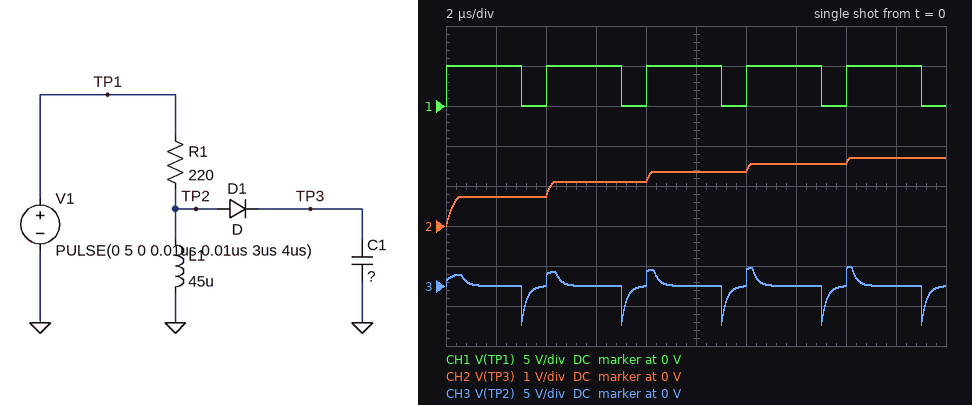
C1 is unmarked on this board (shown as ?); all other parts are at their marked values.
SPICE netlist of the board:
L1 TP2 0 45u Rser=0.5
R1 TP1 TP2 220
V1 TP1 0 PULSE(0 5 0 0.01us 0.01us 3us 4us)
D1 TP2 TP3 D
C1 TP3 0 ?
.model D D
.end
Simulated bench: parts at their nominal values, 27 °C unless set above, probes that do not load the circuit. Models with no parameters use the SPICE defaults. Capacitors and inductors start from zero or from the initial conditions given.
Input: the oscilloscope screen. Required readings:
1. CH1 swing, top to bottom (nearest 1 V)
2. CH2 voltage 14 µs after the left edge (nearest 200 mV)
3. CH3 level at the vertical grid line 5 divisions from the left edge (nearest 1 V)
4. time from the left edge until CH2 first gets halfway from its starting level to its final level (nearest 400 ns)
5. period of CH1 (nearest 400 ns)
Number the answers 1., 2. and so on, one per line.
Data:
1. 5 V
2. 1.6 V
3. 0 V
4. 4.0 µs
5. 4.0 µs
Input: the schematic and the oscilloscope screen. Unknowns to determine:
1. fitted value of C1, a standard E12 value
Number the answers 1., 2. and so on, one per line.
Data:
1. 8.2 nF
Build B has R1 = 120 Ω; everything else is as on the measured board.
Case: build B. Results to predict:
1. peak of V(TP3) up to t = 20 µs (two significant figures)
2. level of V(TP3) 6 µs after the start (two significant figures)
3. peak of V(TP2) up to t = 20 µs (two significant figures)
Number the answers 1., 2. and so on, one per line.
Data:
1. 2.4 V
2. 1.8 V
3. 3.1 V
